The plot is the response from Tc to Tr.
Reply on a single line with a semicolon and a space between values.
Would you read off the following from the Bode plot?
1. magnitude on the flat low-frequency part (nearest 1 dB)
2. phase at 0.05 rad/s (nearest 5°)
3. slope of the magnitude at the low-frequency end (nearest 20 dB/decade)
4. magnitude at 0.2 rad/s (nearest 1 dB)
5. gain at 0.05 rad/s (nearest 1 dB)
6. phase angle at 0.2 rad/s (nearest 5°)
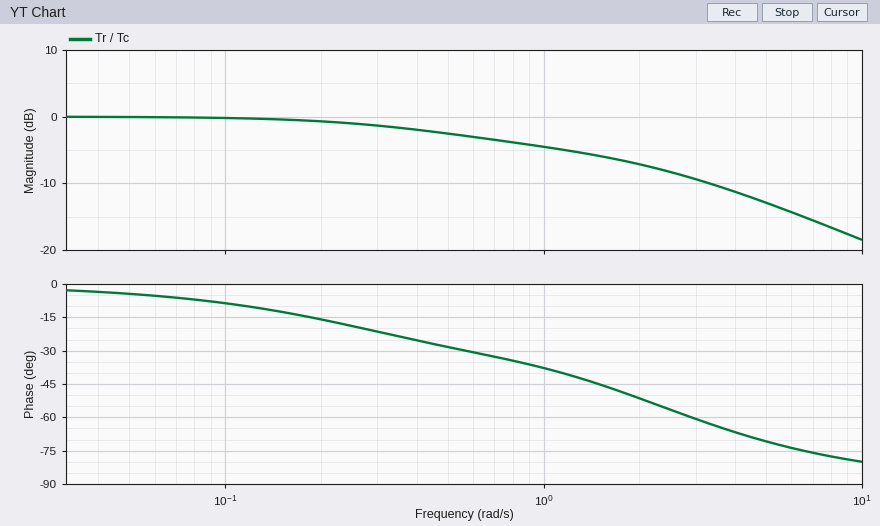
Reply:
0 dB; -5°; 0 dB/decade; -1 dB; 0 dB; -15°
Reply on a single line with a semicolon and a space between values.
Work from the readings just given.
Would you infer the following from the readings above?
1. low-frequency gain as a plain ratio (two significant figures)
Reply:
1.0
